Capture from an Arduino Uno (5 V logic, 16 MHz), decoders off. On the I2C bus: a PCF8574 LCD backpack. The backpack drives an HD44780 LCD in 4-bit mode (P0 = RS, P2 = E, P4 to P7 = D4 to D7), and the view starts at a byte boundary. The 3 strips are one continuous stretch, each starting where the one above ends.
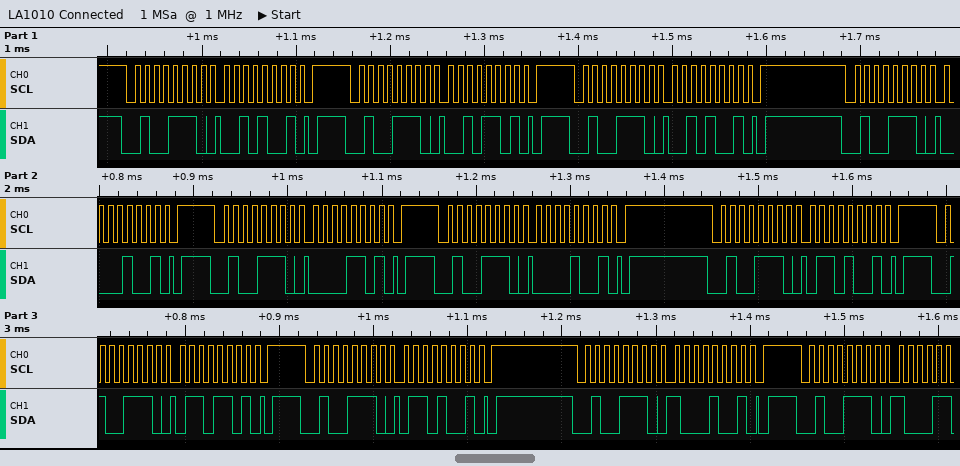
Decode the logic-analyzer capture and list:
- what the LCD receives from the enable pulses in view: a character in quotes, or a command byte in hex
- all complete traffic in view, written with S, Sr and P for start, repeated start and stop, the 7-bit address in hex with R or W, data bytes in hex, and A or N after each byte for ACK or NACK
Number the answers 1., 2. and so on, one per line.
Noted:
1. ' '
2. S 27W A 29 A P S 27W A 2D A P S 27W A 29 A P S 27W A 09 A P S 27W A 0D A P S 27W A 09 A P S 27W A 69 A P S 27W A 6D A P S 27W A 69 A P S 27W A 89 A P S 27W A
